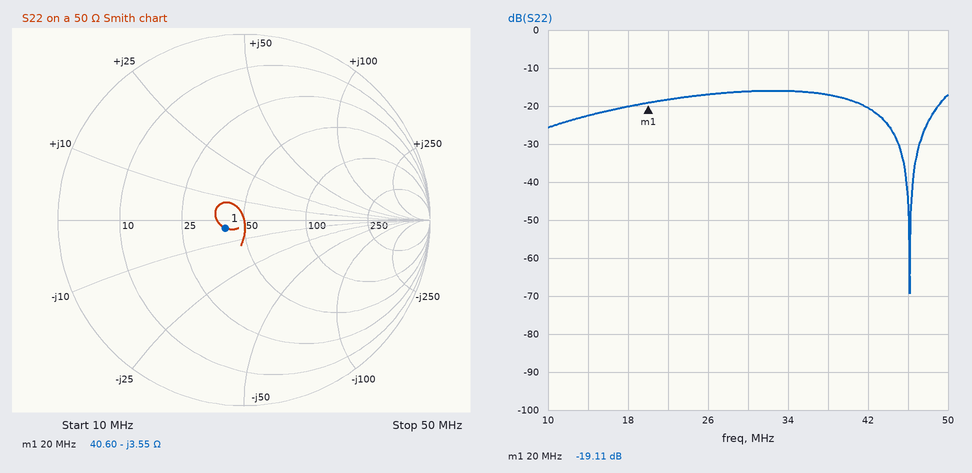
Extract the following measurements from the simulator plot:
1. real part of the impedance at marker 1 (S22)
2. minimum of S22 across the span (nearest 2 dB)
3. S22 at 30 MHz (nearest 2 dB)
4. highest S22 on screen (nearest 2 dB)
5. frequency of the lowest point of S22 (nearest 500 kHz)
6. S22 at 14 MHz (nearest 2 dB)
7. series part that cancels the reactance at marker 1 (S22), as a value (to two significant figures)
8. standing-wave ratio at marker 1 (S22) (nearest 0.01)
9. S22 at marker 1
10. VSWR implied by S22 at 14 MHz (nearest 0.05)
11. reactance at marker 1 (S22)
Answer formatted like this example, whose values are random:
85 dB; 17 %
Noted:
40.60 Ω; -70 dB; -16 dB; -16 dB; 46.0 MHz; -22 dB; 28 nH; 1.25; -19.11 dB; 1.15; -3.55 Ω
